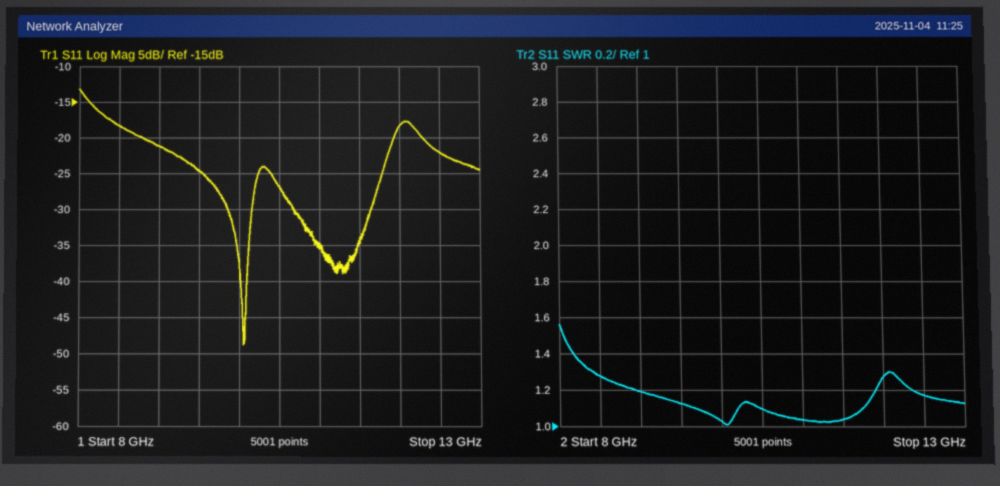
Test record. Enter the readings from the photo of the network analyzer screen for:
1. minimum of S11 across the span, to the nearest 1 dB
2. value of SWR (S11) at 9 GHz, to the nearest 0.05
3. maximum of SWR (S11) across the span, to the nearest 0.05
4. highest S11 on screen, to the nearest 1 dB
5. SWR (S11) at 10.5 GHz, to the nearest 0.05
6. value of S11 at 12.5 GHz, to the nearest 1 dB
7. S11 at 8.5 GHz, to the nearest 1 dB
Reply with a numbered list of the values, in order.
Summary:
1. -49 dB
2. 1.20
3. 1.55
4. -13 dB
5. 1.10
6. -22 dB
7. -18 dB
